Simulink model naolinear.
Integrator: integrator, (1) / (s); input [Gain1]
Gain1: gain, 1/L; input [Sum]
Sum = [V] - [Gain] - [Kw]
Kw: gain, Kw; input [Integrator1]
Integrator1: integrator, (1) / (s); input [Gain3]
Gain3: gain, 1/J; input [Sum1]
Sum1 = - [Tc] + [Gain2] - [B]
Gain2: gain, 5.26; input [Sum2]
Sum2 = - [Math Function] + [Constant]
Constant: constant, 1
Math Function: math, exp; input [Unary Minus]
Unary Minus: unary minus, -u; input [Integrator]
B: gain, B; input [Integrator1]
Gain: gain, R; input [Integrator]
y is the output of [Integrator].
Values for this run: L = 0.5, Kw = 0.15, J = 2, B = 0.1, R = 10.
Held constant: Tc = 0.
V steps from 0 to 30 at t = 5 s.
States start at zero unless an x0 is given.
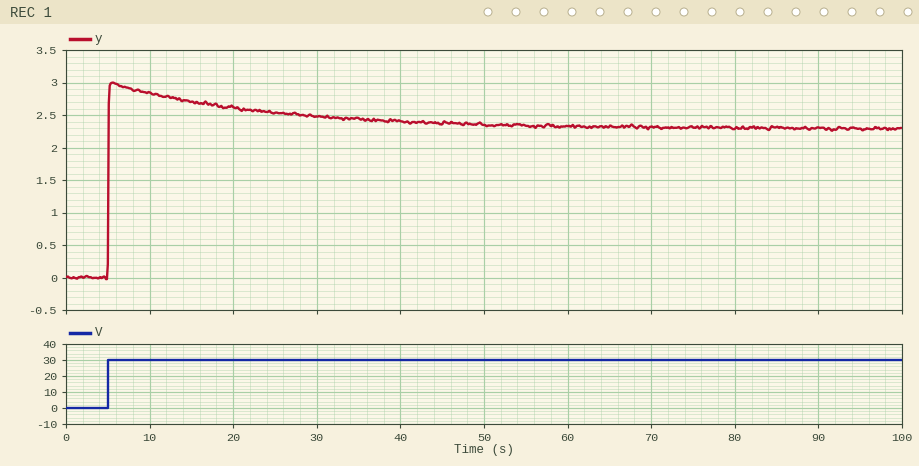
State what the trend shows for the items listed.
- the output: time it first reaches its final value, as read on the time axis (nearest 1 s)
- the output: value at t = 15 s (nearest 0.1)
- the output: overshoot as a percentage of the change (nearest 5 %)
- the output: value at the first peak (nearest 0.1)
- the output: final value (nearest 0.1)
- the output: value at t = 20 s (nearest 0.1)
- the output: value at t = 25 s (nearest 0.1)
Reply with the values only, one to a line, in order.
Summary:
5 s
2.7
30 %
3.0
2.3
2.6
2.5
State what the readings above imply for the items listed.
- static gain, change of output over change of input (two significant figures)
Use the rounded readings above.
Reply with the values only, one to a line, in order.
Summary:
0.077
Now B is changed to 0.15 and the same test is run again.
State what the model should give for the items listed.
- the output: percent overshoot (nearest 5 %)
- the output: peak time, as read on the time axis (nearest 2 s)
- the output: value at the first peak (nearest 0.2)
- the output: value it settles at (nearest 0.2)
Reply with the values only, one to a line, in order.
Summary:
20 %
6 s
3.0
2.6
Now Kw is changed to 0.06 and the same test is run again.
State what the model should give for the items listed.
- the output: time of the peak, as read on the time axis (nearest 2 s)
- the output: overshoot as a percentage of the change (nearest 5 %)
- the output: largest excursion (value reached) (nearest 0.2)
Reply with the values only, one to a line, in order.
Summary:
6 s
10 %
3.0
